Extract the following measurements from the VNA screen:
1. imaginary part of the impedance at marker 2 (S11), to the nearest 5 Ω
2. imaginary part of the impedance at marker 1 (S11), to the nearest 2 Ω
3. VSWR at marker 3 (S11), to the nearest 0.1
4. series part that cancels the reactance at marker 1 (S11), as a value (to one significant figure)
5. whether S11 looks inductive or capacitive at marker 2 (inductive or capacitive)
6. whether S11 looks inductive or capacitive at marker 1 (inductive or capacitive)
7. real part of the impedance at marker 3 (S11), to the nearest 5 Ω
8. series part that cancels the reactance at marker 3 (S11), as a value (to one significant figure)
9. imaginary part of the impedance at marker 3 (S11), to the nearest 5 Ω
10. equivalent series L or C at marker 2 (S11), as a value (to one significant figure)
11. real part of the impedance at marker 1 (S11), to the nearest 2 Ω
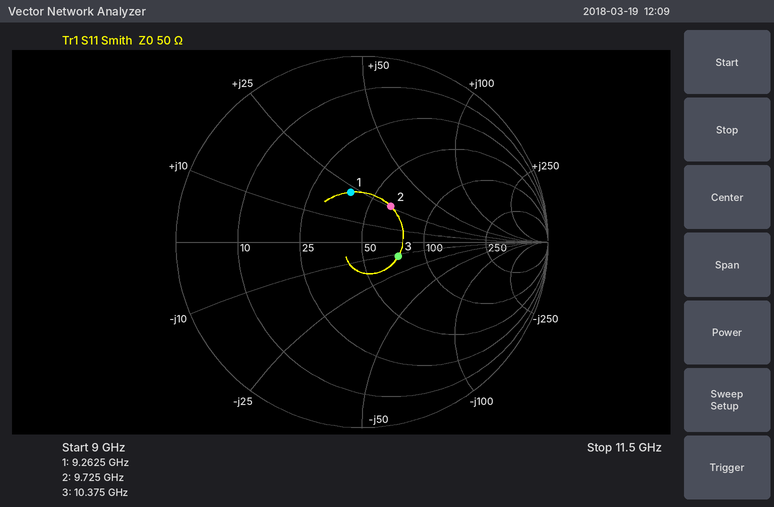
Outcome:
+25 Ω
+22 Ω
1.5
800 fF
inductive
inductive
75 Ω
200 pH
-10 Ω
400 pH
38 Ω
